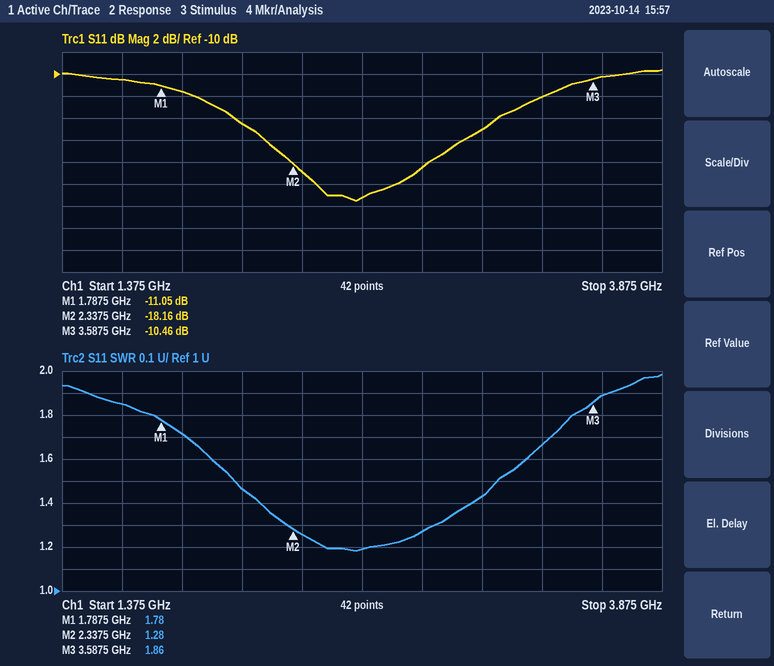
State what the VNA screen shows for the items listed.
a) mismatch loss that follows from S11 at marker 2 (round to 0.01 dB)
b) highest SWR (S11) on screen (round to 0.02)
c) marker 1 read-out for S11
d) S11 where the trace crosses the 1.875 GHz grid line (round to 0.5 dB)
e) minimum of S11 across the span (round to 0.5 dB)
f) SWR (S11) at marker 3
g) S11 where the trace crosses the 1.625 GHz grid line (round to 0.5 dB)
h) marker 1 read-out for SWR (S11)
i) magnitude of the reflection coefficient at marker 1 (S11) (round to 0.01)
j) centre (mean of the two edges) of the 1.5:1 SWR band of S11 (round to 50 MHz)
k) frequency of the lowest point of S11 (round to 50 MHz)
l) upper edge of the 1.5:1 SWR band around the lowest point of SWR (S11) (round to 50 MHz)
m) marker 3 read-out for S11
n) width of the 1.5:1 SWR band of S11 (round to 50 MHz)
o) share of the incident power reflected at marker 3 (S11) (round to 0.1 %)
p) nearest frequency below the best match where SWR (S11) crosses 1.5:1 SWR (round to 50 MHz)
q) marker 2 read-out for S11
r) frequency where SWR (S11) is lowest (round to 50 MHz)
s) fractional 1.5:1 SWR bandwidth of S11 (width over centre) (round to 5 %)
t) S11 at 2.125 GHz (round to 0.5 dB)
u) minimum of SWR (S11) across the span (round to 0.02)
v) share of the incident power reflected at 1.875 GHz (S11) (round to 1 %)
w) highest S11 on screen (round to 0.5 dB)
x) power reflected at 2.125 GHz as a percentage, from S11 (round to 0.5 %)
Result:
0.07 dB
1.98
-11.05 dB
-11.5 dB
-21.5 dB
1.86
-10.5 dB
1.78
0.28
2.65 GHz
2.60 GHz
3.20 GHz
-10.46 dB
1.10 GHz
9.0 %
2.10 GHz
-18.16 dB
2.60 GHz
40 %
-14.5 dB
1.18
7 %
-9.5 dB
3.5 %
